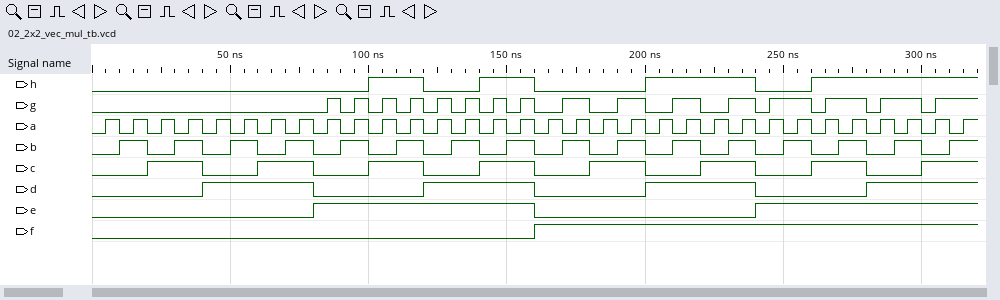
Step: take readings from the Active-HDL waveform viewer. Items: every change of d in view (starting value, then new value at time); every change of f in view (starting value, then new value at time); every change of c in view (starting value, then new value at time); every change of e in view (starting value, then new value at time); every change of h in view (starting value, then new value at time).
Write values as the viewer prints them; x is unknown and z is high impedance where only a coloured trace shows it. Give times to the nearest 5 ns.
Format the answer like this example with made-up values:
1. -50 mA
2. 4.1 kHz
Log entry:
1. 0, 1 at 40 ns, 0 at 80 ns, 1 at 120 ns, 0 at 160 ns, 1 at 200 ns, 0 at 240 ns, 1 at 280 ns
2. 0, 1 at 160 ns
3. 0, 1 at 20 ns, 0 at 40 ns, 1 at 60 ns, 0 at 80 ns, 1 at 100 ns, 0 at 120 ns, 1 at 140 ns, 0 at 160 ns, 1 at 180 ns, 0 at 200 ns, 1 at 220 ns, 0 at 240 ns, 1 at 260 ns, 0 at 280 ns, 1 at 300 ns
4. 0, 1 at 80 ns, 0 at 160 ns, 1 at 240 ns
5. 0, 1 at 100 ns, 0 at 120 ns, 1 at 140 ns, 0 at 160 ns, 1 at 200 ns, 0 at 240 ns, 1 at 260 ns
